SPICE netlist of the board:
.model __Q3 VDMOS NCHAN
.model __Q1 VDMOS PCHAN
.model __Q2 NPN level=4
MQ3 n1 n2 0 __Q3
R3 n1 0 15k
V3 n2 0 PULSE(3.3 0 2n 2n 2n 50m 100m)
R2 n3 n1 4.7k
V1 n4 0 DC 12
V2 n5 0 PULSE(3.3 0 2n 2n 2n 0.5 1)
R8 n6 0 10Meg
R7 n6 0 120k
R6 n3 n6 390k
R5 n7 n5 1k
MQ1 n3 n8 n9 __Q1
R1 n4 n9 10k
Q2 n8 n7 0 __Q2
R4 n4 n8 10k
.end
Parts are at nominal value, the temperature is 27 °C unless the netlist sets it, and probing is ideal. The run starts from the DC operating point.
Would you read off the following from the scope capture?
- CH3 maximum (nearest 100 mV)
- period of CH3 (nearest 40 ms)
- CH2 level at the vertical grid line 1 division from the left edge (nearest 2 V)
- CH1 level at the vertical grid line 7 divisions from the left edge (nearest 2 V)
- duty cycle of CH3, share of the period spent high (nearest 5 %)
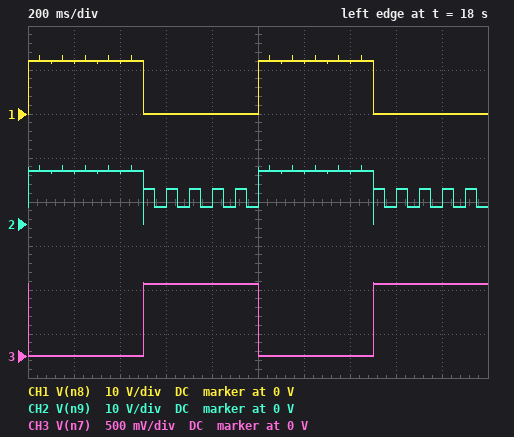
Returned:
800 mV
1.00 s
12 V
12 V
50 %
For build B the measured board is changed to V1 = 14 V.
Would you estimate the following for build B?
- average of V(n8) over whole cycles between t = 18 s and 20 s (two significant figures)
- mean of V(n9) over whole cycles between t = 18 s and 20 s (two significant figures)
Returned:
7.0 V
10 V
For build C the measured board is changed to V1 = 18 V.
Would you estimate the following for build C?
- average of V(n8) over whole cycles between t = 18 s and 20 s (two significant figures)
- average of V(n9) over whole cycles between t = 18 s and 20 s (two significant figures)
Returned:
9.0 V
13 V
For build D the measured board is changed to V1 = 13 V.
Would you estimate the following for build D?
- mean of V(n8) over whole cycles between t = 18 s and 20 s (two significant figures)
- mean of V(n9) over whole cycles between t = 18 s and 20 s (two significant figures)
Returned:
6.5 V
9.7 V
